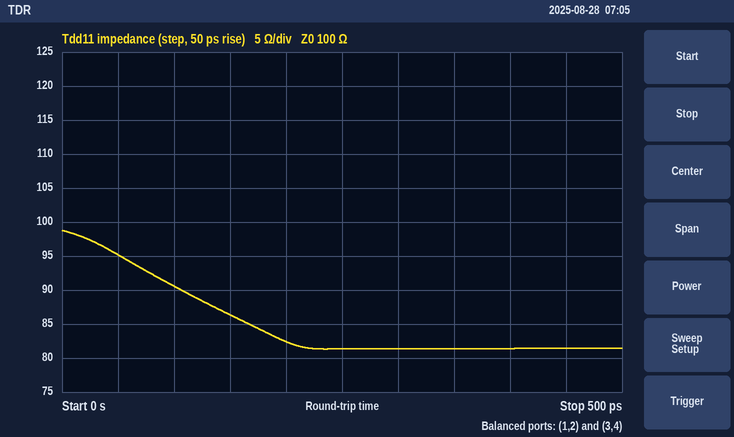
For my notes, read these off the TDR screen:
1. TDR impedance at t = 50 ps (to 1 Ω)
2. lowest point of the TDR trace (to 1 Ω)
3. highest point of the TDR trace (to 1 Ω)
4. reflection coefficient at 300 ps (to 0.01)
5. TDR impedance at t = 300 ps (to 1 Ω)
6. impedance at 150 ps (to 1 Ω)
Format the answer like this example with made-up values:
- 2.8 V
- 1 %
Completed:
- 95 Ω
- 81 Ω
- 99 Ω
- -0.10
- 81 Ω
- 86 Ω
